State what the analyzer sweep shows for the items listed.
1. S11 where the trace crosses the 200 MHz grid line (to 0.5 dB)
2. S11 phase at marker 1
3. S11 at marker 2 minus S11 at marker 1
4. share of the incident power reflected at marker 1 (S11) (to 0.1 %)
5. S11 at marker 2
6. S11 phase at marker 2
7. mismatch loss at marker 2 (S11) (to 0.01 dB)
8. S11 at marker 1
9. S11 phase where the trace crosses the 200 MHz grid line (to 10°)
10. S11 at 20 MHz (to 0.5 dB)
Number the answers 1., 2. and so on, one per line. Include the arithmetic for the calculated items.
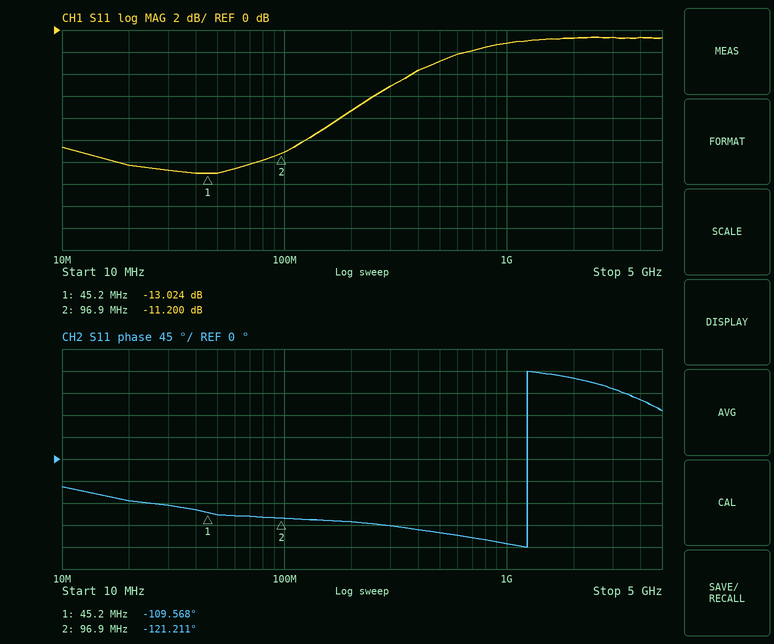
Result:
1. -7.5 dB
2. -109.568°
3. -11.2 − (-13.024) = 1.824 dB
4. 10^(-13.024/10) ≈ 5.0 %
5. -11.200 dB
6. -121.211°
7. −10 log10(1 − 10^(-11.2/10)) ≈ 0.34 dB
8. -13.024 dB
9. -130°
10. -12.5 dB
